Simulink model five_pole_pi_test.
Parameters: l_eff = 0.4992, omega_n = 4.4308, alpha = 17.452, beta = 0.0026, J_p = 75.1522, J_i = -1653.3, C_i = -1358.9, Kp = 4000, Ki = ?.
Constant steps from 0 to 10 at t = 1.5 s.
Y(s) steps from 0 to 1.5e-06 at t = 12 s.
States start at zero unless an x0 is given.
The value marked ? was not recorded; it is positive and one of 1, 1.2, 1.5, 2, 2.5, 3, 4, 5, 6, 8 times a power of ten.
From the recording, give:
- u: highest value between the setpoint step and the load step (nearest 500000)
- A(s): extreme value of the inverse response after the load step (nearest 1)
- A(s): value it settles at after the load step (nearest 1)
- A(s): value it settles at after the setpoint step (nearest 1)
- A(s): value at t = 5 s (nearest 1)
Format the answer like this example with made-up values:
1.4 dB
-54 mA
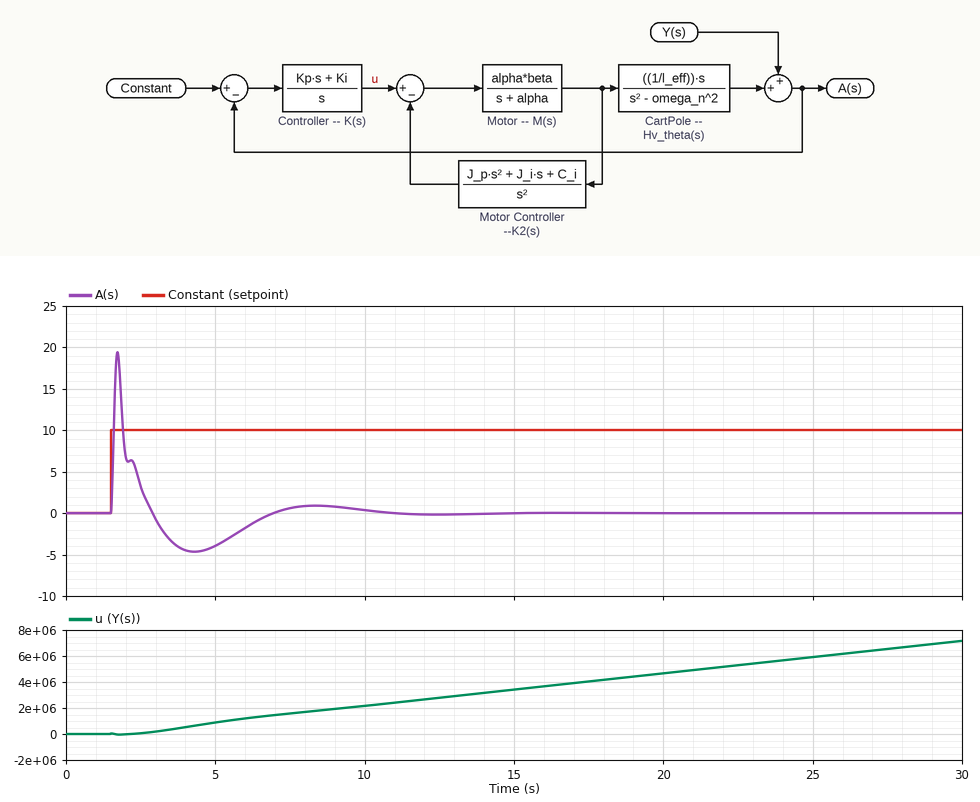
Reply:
2500000
0
0
0
-4
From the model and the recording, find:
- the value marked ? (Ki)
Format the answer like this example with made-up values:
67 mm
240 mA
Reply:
25000
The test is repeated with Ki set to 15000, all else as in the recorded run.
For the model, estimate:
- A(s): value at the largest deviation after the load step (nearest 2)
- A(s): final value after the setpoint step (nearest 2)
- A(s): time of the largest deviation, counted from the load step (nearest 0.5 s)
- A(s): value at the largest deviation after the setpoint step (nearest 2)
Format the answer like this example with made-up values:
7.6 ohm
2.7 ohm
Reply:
0
0
2.0 s
18
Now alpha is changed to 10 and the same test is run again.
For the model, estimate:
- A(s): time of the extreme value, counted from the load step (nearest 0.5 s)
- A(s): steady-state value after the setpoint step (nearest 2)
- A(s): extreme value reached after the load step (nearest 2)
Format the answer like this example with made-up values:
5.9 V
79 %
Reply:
4.5 s
0
0
